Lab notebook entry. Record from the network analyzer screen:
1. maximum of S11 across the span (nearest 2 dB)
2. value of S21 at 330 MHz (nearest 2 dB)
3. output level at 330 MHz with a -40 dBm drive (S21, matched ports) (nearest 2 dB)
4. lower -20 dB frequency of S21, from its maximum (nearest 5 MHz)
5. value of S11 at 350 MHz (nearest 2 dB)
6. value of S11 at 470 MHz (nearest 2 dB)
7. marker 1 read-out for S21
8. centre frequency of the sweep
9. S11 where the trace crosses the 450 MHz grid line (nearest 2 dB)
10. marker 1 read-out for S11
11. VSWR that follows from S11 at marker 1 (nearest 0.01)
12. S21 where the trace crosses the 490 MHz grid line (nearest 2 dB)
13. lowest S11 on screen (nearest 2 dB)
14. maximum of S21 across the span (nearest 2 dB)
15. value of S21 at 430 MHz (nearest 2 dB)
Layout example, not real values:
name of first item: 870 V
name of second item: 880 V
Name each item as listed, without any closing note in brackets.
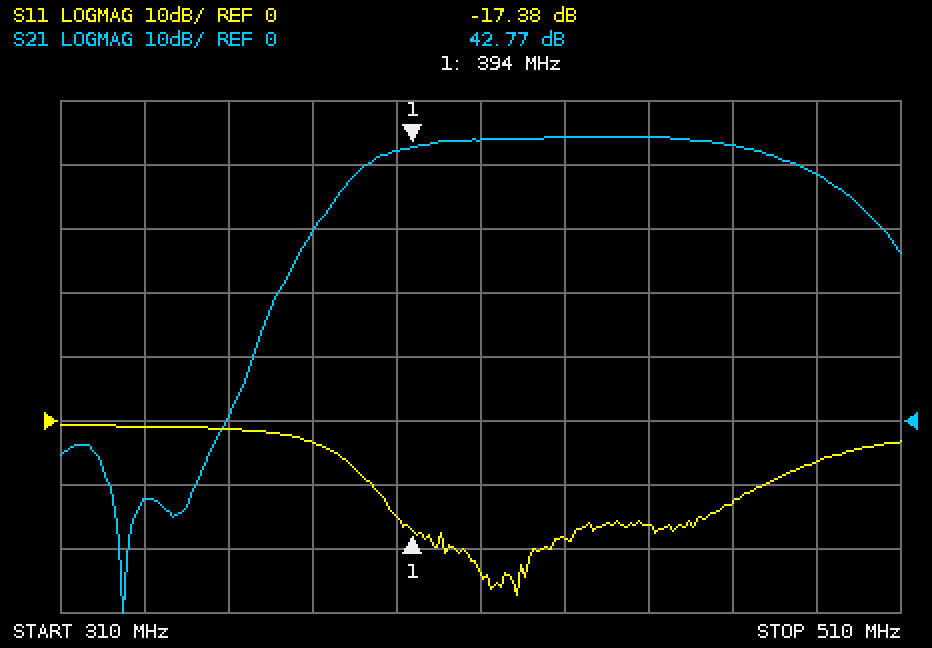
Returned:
maximum of S11 across the span: 0 dB
value of S21 at 330 MHz: -12 dB
output level at 330 MHz with a -40 dBm drive (S21, matched ports): -52 dBm
lower -20 dB frequency of S21, from its maximum: 365 MHz
value of S11 at 350 MHz: -2 dB
value of S11 at 470 MHz: -12 dB
marker 1 read-out for S21: 42.77 dB
centre frequency of the sweep: 410 MHz
S11 where the trace crosses the 450 MHz grid line: -16 dB
marker 1 read-out for S11: -17.38 dB
VSWR that follows from S11 at marker 1: 1.31
S21 where the trace crosses the 490 MHz grid line: 38 dB
lowest S11 on screen: -28 dB
maximum of S21 across the span: 44 dB
value of S21 at 430 MHz: 44 dB
